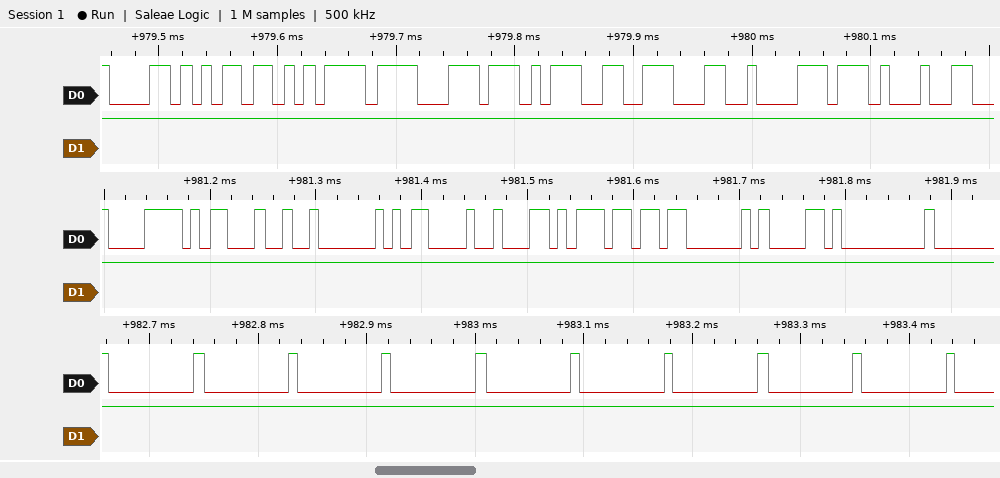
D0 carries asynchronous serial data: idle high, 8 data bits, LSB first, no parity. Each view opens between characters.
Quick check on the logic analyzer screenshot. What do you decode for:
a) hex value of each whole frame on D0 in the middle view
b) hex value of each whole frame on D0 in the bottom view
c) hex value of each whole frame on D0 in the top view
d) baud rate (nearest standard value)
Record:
78, 23, 02, 0D, 62, B7, 03, 61, 00
00, 00, 00, 00, 00, 00, 00, 00, 00
58, 5B, EF, DC, 9D, 8E, C2, 17
115200 baud
